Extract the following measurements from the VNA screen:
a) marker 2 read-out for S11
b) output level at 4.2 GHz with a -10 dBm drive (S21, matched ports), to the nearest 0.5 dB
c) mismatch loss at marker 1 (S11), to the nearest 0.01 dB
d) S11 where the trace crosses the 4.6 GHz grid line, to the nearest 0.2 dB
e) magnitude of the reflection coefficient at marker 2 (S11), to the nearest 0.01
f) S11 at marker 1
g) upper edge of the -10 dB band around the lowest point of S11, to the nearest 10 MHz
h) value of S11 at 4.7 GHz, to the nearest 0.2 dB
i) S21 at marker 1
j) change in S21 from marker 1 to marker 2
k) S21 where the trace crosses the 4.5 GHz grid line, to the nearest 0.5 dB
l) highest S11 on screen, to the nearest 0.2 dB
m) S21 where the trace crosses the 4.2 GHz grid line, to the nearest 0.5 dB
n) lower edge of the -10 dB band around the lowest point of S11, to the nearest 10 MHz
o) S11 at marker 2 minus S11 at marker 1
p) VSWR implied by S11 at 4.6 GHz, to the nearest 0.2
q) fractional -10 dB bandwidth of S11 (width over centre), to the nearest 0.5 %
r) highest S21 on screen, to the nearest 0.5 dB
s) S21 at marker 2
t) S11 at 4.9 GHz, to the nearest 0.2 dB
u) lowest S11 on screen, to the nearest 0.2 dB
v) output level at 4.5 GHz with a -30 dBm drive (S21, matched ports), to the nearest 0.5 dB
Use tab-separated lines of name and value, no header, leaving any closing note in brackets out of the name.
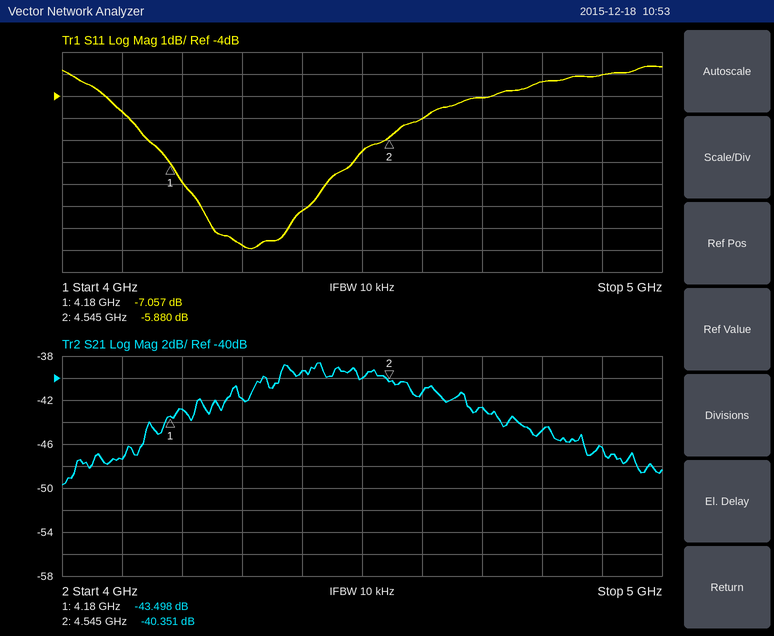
marker 2 read-out for S11	-5.880 dB
output level at 4.2 GHz with a -10 dBm drive (S21, matched ports), to the nearest 0.5 dB	-53.0 dBm
mismatch loss at marker 1 (S11), to the nearest 0.01 dB	0.95 dB
S11 where the trace crosses the 4.6 GHz grid line, to the nearest 0.2 dB	-5.0 dB
magnitude of the reflection coefficient at marker 2 (S11), to the nearest 0.01	0.51
S11 at marker 1	-7.057 dB
upper edge of the -10 dB band around the lowest point of S11, to the nearest 10 MHz	4.38 GHz
value of S11 at 4.7 GHz, to the nearest 0.2 dB	-4.0 dB
S21 at marker 1	-43.498 dB
change in S21 from marker 1 to marker 2	3.147 dB
S21 where the trace crosses the 4.5 GHz grid line, to the nearest 0.5 dB	-40.0 dB
highest S11 on screen, to the nearest 0.2 dB	-2.6 dB
S21 where the trace crosses the 4.2 GHz grid line, to the nearest 0.5 dB	-43.0 dB
lower edge of the -10 dB band around the lowest point of S11, to the nearest 10 MHz	4.25 GHz
S11 at marker 2 minus S11 at marker 1	1.177 dB
VSWR implied by S11 at 4.6 GHz, to the nearest 0.2	3.6
fractional -10 dB bandwidth of S11 (width over centre), to the nearest 0.5 %	3.0 %
highest S21 on screen, to the nearest 0.5 dB	-38.5 dB
S21 at marker 2	-40.351 dB
S11 at 4.9 GHz, to the nearest 0.2 dB	-3.0 dB
lowest S11 on screen, to the nearest 0.2 dB	-11.0 dB
output level at 4.5 GHz with a -30 dBm drive (S21, matched ports), to the nearest 0.5 dB	-70.0 dBm
